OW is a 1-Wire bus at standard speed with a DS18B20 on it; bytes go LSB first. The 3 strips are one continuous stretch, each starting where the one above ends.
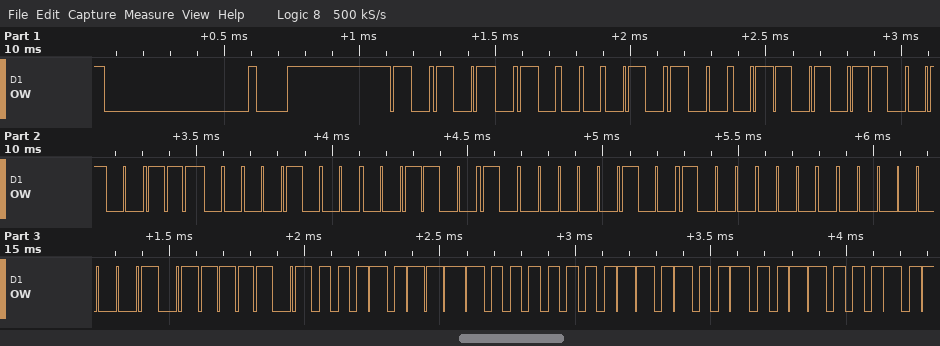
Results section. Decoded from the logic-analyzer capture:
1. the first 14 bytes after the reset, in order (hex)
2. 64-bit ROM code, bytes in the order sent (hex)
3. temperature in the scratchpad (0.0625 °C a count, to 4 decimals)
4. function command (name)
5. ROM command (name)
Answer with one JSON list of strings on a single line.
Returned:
["55 28 D6 E4 10 4C 20 01 80 BE E8 01 4B 46", "28 D6 E4 10 4C 20 01 80", "30.5000 °C", "Read Scratchpad", "Match ROM"]
